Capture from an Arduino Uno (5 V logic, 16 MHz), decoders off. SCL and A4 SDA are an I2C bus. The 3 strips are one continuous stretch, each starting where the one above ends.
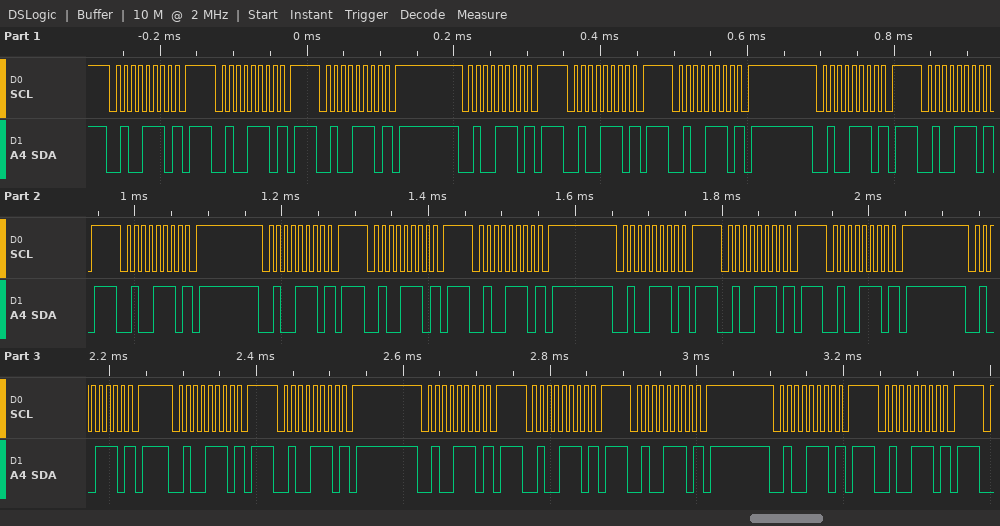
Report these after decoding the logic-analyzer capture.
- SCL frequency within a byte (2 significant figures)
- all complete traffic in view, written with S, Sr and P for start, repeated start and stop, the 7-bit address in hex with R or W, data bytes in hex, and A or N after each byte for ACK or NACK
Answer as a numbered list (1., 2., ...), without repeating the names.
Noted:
1. 100 kHz
2. S 27W N P S 27W N P S 27W N P S 27W N P S 27W N P S 27W N P S 27W N P S 27W N P S 27W N P S 27W N P S 27W N P S 27W N P S 27W N P S 27W N P S 27W N P S 27W N P S 27W N P S 27W N P S 27W N P S 27W N P S 27W N P S 27W N P S 27W N P
